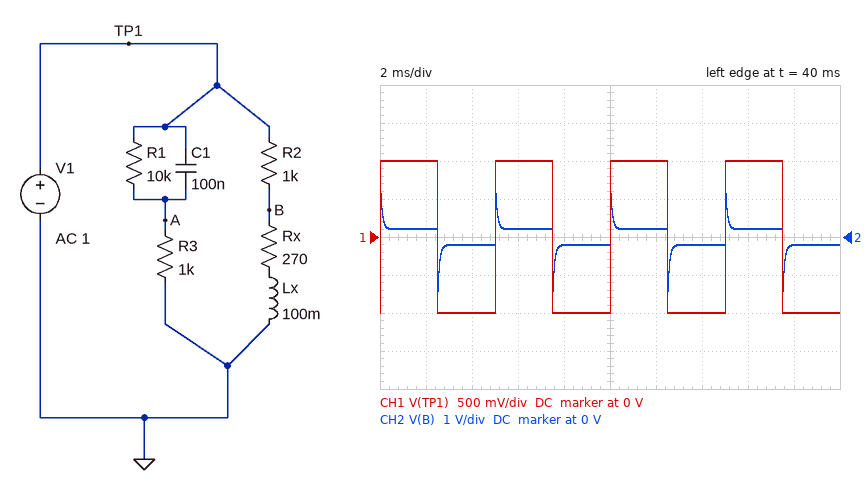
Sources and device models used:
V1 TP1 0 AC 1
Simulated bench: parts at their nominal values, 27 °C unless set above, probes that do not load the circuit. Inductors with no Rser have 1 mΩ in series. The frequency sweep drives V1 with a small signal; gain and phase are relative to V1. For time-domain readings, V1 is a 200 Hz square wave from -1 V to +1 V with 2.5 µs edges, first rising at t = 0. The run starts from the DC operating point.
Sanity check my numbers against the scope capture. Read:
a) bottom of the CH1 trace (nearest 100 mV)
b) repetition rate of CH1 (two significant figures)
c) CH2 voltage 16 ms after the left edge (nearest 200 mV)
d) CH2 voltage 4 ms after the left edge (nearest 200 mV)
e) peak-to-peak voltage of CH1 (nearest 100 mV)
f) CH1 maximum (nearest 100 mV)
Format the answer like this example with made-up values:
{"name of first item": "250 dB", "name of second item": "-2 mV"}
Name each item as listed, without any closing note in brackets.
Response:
{"bottom of the CH1 trace": "-1.0 V", "repetition rate of CH1": "200 Hz", "CH2 voltage 16 ms after the left edge": "200 mV", "CH2 voltage 4 ms after the left edge": "-200 mV", "peak-to-peak voltage of CH1": "2.0 V", "CH1 maximum": "1.0 V"}
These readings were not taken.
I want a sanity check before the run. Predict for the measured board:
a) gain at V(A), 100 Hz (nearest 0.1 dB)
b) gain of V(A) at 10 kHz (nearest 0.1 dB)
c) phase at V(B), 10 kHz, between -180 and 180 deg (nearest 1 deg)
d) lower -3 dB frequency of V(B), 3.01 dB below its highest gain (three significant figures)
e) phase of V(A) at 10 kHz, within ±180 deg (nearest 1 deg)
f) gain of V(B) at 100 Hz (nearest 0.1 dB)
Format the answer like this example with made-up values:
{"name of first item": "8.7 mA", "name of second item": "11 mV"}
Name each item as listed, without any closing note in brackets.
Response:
{"gain at V(A), 100 Hz": "-19.4 dB", "gain of V(A) at 10 kHz": "-0.1 dB", "phase at V(B), 10 kHz, between -180 and 180 deg": "9 deg", "lower -3 dB frequency of V(B), 3.01 dB below its highest gain": "1.93 kHz", "phase of V(A) at 10 kHz, within ±180 deg": "9 deg", "gain of V(B) at 100 Hz": "-13.2 dB"}
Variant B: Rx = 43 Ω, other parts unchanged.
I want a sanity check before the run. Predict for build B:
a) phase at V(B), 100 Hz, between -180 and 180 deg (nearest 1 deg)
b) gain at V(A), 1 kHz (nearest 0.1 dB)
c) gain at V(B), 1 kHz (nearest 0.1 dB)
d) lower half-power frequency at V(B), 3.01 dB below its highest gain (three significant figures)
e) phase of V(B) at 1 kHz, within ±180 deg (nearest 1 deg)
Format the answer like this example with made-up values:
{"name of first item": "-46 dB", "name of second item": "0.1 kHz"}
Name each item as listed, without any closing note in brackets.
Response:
{"phase at V(B), 100 Hz, between -180 and 180 deg": "52 deg", "gain at V(A), 1 kHz": "-6.0 dB", "gain at V(B), 1 kHz": "-5.7 dB", "lower half-power frequency at V(B), 3.01 dB below its highest gain": "1.66 kHz", "phase of V(B) at 1 kHz, within ±180 deg": "55 deg"}
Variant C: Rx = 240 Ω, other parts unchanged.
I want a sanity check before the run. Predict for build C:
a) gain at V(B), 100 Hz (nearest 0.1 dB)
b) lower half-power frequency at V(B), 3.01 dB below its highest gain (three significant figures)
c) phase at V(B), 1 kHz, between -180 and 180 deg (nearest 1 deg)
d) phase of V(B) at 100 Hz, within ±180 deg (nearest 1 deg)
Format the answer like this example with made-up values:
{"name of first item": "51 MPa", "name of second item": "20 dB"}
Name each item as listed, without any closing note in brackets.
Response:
{"gain at V(B), 100 Hz": "-14.0 dB", "lower half-power frequency at V(B), 3.01 dB below its highest gain": "1.90 kHz", "phase at V(B), 1 kHz, between -180 and 180 deg": "42 deg", "phase of V(B) at 100 Hz, within ±180 deg": "12 deg"}
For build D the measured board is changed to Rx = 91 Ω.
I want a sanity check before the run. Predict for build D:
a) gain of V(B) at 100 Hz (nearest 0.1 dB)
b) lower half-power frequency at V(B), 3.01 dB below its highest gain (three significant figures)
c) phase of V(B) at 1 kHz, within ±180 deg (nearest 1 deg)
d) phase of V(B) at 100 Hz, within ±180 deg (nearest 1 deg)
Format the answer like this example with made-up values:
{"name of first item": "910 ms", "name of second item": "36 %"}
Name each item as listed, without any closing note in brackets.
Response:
{"gain of V(B) at 100 Hz": "-19.9 dB", "lower half-power frequency at V(B), 3.01 dB below its highest gain": "1.72 kHz", "phase of V(B) at 1 kHz, within ±180 deg": "52 deg", "phase of V(B) at 100 Hz, within ±180 deg": "31 deg"}
